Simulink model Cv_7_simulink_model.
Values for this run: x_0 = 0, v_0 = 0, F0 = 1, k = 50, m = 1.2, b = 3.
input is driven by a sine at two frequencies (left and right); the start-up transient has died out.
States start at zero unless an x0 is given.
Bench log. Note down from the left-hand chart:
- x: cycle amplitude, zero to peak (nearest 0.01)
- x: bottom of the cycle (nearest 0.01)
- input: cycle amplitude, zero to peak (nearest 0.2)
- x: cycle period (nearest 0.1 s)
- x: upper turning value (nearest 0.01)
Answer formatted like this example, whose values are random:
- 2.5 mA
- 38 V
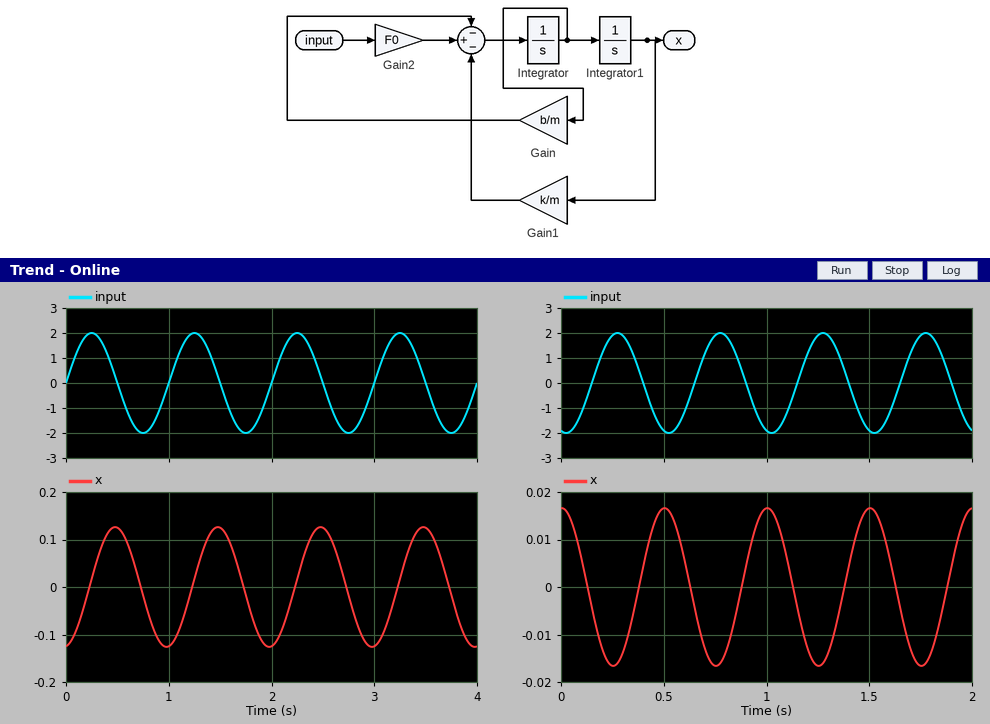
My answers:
- 0.13
- -0.13
- 2.0
- 1.0 s
- 0.13
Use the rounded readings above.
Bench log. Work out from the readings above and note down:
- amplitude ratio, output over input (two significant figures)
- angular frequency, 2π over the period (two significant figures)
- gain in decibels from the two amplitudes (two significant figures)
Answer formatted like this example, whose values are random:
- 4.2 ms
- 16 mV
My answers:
- 0.065
- 6.3 rad/s
- -24 dB
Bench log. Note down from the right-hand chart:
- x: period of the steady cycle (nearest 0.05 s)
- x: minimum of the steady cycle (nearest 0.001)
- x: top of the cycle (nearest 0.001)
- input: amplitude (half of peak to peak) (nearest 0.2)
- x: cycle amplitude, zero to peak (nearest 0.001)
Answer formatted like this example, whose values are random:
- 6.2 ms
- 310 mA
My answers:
- 0.50 s
- -0.017
- 0.017
- 2.0
- 0.017
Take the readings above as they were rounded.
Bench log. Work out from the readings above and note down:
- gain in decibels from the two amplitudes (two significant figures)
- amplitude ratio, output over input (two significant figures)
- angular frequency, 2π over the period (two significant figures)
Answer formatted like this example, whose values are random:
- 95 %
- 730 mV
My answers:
- -41 dB
- 0.0085
- 13 rad/s
